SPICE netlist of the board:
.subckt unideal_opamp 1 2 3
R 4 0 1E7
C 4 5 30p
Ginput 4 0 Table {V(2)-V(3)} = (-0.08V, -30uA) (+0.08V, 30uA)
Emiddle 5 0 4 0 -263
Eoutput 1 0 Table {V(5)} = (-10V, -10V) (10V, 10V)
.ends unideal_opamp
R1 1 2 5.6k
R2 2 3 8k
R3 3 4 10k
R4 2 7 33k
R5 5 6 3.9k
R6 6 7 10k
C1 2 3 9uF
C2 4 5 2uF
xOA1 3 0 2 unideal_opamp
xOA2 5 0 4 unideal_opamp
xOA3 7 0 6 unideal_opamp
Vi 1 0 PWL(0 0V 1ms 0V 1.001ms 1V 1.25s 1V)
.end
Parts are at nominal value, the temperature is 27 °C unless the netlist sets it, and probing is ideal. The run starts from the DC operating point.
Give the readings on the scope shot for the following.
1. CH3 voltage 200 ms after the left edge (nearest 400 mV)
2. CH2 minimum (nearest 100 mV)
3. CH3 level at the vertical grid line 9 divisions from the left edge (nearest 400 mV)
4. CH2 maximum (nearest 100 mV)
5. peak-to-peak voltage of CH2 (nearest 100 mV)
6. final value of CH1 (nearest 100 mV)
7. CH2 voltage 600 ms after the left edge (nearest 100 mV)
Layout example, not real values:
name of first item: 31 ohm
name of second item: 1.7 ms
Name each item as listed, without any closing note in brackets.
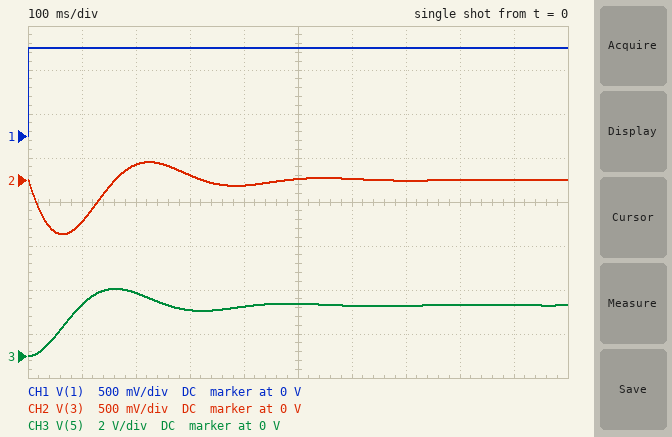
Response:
CH3 voltage 200 ms after the left edge: 2.8 V
CH2 minimum: -600 mV
CH3 level at the vertical grid line 9 divisions from the left edge: 2.4 V
CH2 maximum: 200 mV
peak-to-peak voltage of CH2: 800 mV
final value of CH1: 1.0 V
CH2 voltage 600 ms after the left edge: 0 V
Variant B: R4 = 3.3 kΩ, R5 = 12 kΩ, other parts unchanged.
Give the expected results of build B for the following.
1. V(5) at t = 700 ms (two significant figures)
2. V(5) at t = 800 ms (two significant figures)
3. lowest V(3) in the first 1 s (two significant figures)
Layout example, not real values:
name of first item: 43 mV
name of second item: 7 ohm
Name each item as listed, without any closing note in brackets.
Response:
V(5) at t = 700 ms: 700 mV
V(5) at t = 800 ms: 710 mV
lowest V(3) in the first 1 s: -410 mV
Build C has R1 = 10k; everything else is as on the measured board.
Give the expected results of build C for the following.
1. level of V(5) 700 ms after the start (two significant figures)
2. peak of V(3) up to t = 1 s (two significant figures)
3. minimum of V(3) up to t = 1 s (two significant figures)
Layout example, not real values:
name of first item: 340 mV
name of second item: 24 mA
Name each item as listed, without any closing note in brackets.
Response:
level of V(5) 700 ms after the start: 1.3 V
peak of V(3) up to t = 1 s: 110 mV
minimum of V(3) up to t = 1 s: -350 mV
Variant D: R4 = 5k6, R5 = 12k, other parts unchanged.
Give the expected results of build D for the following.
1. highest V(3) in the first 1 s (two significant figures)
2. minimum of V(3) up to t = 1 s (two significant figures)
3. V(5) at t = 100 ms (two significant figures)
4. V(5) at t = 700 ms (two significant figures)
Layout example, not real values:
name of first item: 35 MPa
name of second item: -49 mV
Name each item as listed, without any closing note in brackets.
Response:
highest V(3) in the first 1 s: 230 mV
minimum of V(3) up to t = 1 s: -500 mV
V(5) at t = 100 ms: 1.7 V
V(5) at t = 700 ms: 1.2 V
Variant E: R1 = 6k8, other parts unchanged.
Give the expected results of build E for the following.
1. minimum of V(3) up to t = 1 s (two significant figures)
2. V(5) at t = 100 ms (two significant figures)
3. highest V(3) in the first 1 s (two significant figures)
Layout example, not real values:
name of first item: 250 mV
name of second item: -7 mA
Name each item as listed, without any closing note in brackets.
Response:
minimum of V(3) up to t = 1 s: -510 mV
V(5) at t = 100 ms: 1.9 V
highest V(3) in the first 1 s: 170 mV
